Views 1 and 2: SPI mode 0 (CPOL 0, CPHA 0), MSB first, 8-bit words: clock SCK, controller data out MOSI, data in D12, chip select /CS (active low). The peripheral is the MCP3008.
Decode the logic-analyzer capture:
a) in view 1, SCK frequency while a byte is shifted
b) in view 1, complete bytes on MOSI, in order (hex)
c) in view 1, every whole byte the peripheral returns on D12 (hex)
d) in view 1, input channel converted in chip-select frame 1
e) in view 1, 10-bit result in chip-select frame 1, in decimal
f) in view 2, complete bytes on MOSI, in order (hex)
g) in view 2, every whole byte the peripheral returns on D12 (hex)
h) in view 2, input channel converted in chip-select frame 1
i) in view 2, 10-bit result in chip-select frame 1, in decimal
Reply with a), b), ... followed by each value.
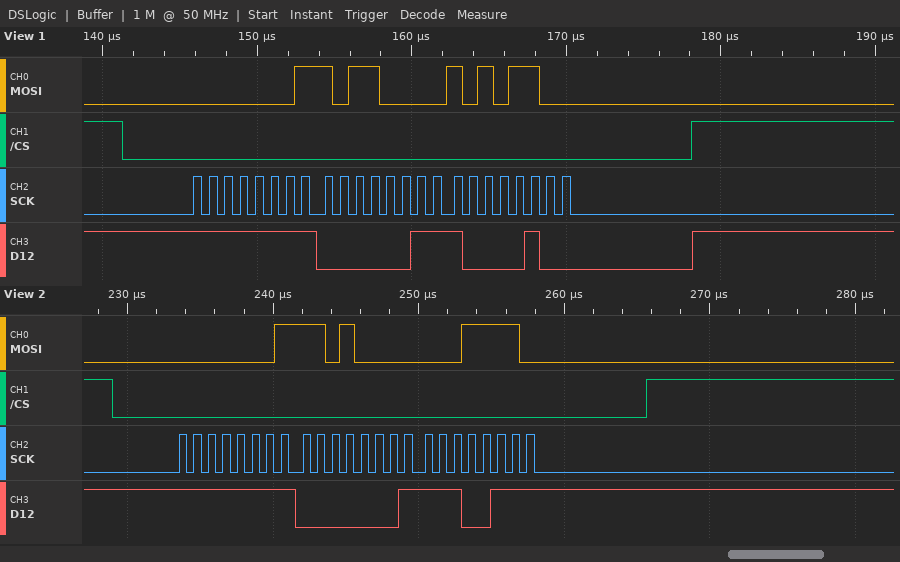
a) 1 MHz
b) 01 B0 AC
c) FF 03 84
d) 3
e) 900
f) 01 D0 1E
g) FF 01 E7
h) 5
i) 487
